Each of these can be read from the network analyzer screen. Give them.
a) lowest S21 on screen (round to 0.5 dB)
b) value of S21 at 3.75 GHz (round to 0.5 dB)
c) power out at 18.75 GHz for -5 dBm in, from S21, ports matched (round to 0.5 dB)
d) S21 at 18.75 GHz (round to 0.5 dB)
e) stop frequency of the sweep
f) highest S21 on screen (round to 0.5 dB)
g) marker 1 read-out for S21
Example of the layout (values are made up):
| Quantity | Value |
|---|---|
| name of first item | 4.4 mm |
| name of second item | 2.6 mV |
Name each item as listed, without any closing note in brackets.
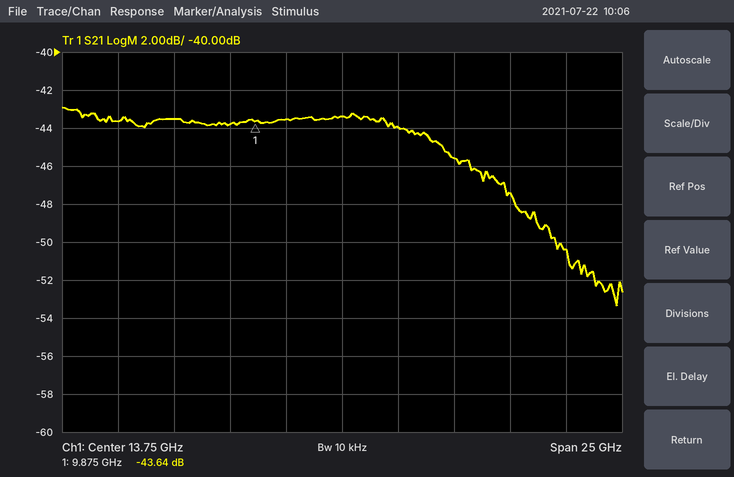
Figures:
| Quantity | Value |
|---|---|
| lowest S21 on screen | -53.5 dB |
| value of S21 at 3.75 GHz | -43.5 dB |
| power out at 18.75 GHz for -5 dBm in, from S21, ports matched | -50.5 dBm |
| S21 at 18.75 GHz | -45.5 dB |
| stop frequency of the sweep | 26.25 GHz |
| highest S21 on screen | -43.0 dB |
| marker 1 read-out for S21 | -43.64 dB |
